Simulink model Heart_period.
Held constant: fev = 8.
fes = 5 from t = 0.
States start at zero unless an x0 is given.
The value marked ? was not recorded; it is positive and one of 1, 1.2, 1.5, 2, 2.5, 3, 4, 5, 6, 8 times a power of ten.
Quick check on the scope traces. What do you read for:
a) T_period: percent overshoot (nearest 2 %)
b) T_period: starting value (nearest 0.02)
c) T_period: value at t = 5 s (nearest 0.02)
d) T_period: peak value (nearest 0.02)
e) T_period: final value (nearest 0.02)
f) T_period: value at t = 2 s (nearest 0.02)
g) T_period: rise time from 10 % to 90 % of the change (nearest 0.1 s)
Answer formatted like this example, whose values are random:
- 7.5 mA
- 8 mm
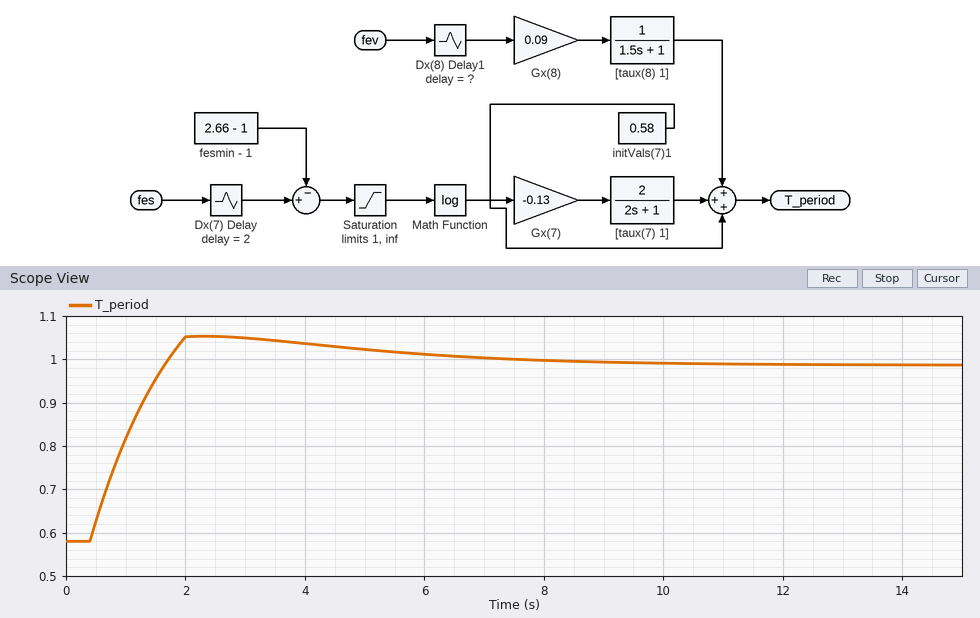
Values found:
- 16 %
- 0.58
- 1.02
- 1.06
- 0.98
- 1.06
- 1.0 s
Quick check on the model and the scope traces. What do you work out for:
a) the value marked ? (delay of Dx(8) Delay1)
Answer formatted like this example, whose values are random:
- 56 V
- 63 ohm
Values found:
- 0.4
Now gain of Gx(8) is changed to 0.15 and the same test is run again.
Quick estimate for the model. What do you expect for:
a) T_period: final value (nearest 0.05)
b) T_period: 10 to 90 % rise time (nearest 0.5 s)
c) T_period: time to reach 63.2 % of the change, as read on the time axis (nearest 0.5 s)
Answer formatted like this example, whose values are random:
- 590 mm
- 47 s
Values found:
- 1.45
- 1.5 s
- 1.5 s
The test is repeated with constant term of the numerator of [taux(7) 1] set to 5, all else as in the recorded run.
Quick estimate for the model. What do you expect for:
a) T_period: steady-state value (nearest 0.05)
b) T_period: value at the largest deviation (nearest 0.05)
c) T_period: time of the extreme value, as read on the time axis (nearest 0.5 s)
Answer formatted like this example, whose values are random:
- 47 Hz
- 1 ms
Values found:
- 0.50
- 1.05
- 2.0 s
